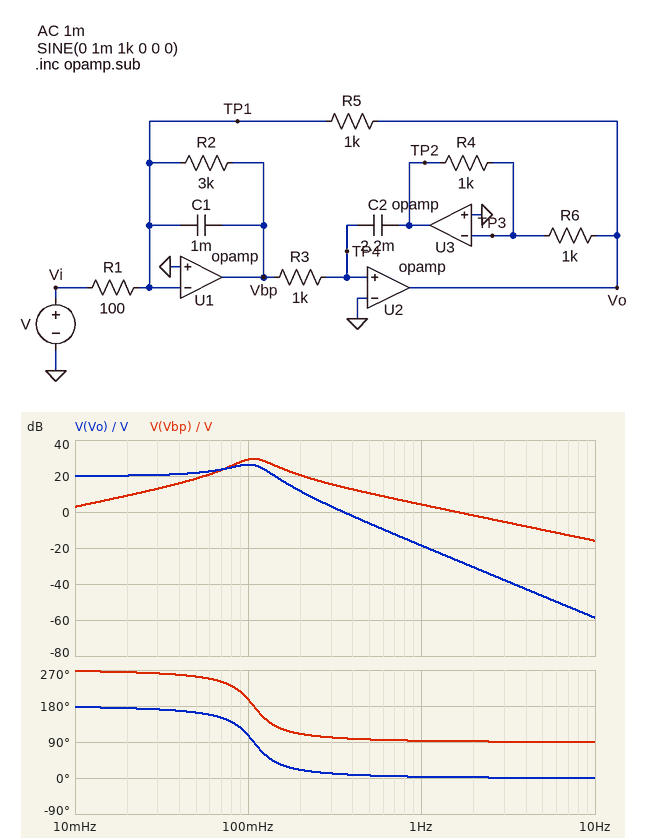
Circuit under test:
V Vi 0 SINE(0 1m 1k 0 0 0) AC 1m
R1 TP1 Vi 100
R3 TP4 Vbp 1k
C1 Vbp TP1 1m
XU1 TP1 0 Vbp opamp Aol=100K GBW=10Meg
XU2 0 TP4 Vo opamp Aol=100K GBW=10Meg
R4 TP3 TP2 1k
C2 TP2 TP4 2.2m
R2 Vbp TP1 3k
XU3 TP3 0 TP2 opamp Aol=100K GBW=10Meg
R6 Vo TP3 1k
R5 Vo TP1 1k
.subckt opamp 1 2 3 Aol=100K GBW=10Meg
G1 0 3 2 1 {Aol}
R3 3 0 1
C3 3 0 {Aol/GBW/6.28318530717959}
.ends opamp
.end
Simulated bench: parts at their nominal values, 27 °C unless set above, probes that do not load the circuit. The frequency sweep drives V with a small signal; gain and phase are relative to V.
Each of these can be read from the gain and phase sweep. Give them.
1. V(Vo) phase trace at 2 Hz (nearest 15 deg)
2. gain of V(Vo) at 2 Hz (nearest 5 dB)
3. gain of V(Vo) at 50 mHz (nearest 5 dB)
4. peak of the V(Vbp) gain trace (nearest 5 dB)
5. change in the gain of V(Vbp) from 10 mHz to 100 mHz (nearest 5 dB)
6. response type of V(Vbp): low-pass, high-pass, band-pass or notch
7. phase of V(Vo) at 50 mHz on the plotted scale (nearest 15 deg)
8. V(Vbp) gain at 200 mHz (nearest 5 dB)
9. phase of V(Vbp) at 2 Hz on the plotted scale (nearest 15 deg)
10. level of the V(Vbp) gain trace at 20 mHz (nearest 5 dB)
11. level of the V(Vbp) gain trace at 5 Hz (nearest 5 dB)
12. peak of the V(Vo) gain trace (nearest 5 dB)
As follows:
0 deg
-30 dB
20 dB
30 dB
25 dB
band-pass
165 deg
20 dB
90 deg
10 dB
-10 dB
25 dB
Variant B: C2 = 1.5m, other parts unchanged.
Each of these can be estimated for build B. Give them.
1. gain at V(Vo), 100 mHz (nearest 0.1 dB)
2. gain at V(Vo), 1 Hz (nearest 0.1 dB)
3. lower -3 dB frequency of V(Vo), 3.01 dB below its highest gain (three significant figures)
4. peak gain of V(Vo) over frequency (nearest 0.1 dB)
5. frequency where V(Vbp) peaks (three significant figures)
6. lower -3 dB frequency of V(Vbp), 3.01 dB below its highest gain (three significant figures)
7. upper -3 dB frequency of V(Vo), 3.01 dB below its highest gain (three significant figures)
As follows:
25.8 dB
-15.3 dB
93.4 mHz
28.0 dB
130 mHz
106 mHz
149 mHz
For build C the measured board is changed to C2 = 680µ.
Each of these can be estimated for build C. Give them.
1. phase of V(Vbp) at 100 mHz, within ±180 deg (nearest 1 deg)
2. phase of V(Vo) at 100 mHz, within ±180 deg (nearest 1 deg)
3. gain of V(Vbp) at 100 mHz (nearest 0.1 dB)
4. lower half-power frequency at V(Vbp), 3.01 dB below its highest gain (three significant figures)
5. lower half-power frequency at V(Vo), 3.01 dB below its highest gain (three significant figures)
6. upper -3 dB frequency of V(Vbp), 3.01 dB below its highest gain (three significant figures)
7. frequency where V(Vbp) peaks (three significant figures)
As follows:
-101 deg
169 deg
15.2 dB
168 mHz
160 mHz
221 mHz
193 mHz
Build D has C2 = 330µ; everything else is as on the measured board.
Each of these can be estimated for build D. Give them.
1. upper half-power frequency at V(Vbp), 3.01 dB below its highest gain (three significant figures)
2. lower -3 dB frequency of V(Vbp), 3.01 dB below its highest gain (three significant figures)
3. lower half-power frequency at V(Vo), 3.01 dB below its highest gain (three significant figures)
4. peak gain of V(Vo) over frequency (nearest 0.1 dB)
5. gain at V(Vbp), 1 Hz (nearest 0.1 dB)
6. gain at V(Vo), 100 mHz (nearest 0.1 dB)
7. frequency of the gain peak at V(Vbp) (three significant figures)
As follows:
305 mHz
252 mHz
246 mHz
34.4 dB
4.7 dB
21.2 dB
277 mHz
